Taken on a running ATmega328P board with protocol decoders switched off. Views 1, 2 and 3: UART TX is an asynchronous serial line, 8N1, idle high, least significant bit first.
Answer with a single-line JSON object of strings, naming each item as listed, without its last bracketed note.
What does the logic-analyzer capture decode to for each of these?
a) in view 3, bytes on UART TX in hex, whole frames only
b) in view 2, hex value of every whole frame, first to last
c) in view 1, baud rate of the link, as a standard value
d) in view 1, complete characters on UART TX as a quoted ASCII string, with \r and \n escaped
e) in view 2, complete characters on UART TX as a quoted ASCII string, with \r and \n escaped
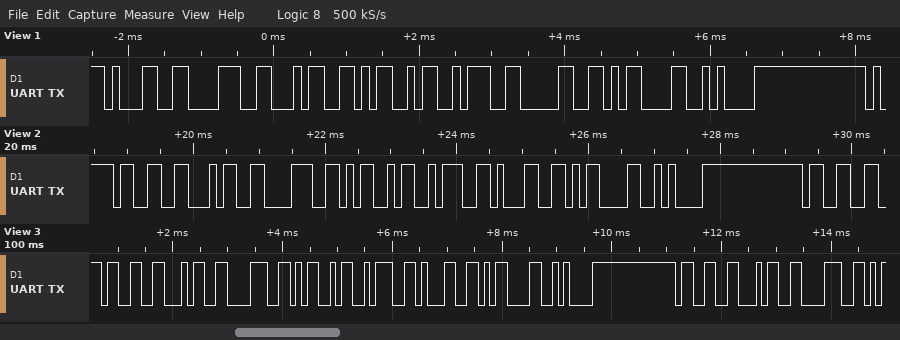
{"in view 3, bytes on UART TX in hex, whole frames only": "33 34 38 4D 3A 31 0D 0A 33 34 38", "in view 2, hex value of every whole frame, first to last": "33 34 38 4D 3A 31 0D 0A 33", "in view 1, baud rate of the link, as a standard value": "9600 baud", "in view 1, complete characters on UART TX as a quoted ASCII string, with \\r and \\n escaped": "\"184M:0\\r\\n\"", "in view 2, complete characters on UART TX as a quoted ASCII string, with \\r and \\n escaped": "\"348M:1\\r\\n3\""}
